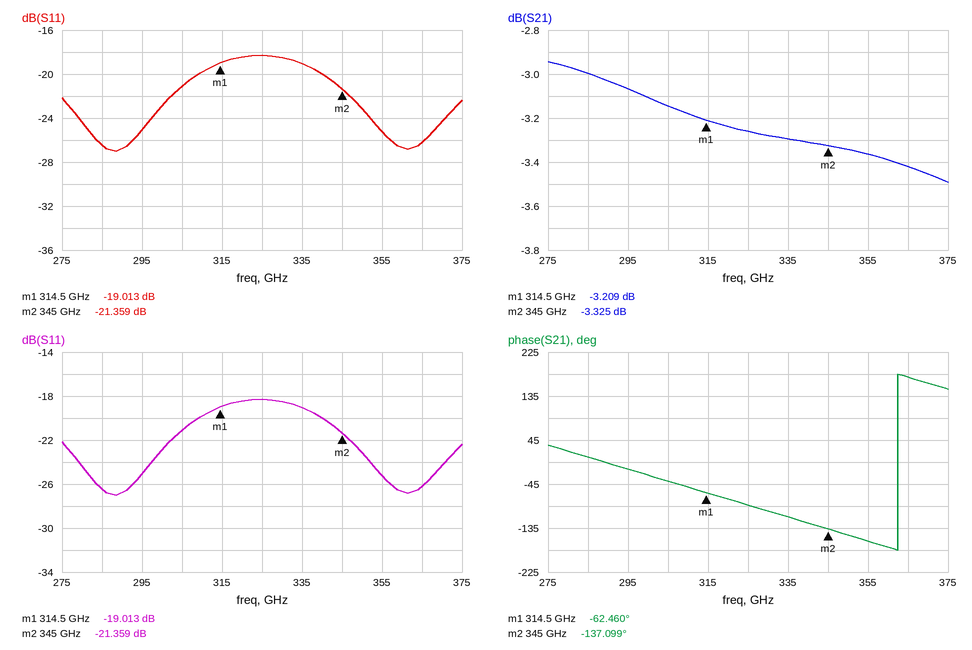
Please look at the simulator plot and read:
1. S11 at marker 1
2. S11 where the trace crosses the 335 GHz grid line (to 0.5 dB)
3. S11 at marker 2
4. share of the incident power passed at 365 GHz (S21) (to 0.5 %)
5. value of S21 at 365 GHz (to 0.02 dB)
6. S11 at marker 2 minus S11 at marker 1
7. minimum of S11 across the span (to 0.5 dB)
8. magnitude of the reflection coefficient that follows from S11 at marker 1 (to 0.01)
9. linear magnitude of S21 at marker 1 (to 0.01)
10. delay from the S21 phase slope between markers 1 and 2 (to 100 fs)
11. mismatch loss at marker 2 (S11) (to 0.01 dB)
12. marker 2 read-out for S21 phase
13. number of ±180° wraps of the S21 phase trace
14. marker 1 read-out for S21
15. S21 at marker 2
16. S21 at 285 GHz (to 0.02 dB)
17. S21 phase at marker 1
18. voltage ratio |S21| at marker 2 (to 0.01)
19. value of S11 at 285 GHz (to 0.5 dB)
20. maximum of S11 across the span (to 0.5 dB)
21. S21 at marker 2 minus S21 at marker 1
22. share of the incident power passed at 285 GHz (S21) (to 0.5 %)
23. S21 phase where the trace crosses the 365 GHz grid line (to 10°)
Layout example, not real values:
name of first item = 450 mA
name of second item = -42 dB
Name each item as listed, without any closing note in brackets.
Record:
S11 at marker 1 = -19.013 dB
S11 where the trace crosses the 335 GHz grid line = -19.0 dB
S11 at marker 2 = -21.359 dB
share of the incident power passed at 365 GHz (S21) = 45.5 %
value of S21 at 365 GHz = -3.42 dB
S11 at marker 2 minus S11 at marker 1 = -2.346 dB
minimum of S11 across the span = -27.0 dB
magnitude of the reflection coefficient that follows from S11 at marker 1 = 0.11
linear magnitude of S21 at marker 1 = 0.69
delay from the S21 phase slope between markers 1 and 2 = 6.8 ps
mismatch loss at marker 2 (S11) = 0.03 dB
marker 2 read-out for S21 phase = -137.099°
number of ±180° wraps of the S21 phase trace = 1
marker 1 read-out for S21 = -3.209 dB
S21 at marker 2 = -3.325 dB
S21 at 285 GHz = -3.00 dB
S21 phase at marker 1 = -62.460°
voltage ratio |S21| at marker 2 = 0.68
value of S11 at 285 GHz = -26.5 dB
maximum of S11 across the span = -18.5 dB
S21 at marker 2 minus S21 at marker 1 = -0.116 dB
share of the incident power passed at 285 GHz (S21) = 50.0 %
S21 phase where the trace crosses the 365 GHz grid line = 170°
